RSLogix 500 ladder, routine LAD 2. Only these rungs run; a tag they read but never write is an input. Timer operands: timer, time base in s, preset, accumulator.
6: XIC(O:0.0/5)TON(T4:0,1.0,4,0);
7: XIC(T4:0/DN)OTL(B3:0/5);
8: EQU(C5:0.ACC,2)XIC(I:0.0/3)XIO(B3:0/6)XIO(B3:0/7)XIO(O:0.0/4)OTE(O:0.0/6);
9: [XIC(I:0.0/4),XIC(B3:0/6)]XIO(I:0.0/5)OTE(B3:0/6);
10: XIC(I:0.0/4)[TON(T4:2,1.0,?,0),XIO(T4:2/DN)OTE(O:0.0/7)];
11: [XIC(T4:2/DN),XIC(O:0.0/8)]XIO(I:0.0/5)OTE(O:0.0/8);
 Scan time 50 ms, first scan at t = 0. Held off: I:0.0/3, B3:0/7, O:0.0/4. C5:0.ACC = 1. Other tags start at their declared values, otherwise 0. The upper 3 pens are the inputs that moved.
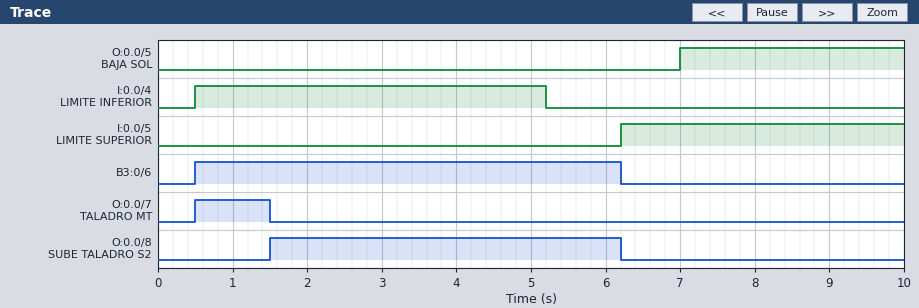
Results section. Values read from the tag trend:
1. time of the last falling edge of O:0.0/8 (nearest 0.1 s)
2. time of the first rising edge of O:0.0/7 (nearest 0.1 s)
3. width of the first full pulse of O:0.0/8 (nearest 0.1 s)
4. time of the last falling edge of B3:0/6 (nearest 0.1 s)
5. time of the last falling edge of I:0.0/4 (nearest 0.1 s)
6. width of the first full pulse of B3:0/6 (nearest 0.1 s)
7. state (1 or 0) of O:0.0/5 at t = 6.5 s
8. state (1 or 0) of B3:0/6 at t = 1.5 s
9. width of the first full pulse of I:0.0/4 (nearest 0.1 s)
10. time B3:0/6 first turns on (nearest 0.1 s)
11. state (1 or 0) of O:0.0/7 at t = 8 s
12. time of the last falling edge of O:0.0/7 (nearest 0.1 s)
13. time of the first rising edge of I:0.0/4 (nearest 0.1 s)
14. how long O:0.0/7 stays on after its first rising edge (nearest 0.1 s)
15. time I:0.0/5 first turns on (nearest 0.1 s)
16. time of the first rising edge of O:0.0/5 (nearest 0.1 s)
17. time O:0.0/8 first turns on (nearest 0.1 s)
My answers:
6.2 s
0.5 s
4.7 s
6.2 s
5.2 s
5.7 s
0
1
4.7 s
0.5 s
0
1.5 s
0.5 s
1.0 s
6.2 s
7.0 s
1.5 s
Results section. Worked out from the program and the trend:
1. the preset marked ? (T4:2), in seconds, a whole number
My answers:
1 s
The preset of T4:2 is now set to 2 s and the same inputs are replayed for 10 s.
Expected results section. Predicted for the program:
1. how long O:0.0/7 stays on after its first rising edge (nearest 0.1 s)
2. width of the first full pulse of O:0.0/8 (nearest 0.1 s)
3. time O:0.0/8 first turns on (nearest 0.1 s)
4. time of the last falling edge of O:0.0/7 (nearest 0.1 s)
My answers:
2.0 s
3.7 s
2.5 s
2.5 s
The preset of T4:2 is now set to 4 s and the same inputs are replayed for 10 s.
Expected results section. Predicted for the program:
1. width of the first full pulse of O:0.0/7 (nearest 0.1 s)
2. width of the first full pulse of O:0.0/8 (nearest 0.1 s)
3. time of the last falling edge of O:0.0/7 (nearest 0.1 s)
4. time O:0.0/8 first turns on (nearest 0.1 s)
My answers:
4.0 s
1.7 s
4.5 s
4.5 s
